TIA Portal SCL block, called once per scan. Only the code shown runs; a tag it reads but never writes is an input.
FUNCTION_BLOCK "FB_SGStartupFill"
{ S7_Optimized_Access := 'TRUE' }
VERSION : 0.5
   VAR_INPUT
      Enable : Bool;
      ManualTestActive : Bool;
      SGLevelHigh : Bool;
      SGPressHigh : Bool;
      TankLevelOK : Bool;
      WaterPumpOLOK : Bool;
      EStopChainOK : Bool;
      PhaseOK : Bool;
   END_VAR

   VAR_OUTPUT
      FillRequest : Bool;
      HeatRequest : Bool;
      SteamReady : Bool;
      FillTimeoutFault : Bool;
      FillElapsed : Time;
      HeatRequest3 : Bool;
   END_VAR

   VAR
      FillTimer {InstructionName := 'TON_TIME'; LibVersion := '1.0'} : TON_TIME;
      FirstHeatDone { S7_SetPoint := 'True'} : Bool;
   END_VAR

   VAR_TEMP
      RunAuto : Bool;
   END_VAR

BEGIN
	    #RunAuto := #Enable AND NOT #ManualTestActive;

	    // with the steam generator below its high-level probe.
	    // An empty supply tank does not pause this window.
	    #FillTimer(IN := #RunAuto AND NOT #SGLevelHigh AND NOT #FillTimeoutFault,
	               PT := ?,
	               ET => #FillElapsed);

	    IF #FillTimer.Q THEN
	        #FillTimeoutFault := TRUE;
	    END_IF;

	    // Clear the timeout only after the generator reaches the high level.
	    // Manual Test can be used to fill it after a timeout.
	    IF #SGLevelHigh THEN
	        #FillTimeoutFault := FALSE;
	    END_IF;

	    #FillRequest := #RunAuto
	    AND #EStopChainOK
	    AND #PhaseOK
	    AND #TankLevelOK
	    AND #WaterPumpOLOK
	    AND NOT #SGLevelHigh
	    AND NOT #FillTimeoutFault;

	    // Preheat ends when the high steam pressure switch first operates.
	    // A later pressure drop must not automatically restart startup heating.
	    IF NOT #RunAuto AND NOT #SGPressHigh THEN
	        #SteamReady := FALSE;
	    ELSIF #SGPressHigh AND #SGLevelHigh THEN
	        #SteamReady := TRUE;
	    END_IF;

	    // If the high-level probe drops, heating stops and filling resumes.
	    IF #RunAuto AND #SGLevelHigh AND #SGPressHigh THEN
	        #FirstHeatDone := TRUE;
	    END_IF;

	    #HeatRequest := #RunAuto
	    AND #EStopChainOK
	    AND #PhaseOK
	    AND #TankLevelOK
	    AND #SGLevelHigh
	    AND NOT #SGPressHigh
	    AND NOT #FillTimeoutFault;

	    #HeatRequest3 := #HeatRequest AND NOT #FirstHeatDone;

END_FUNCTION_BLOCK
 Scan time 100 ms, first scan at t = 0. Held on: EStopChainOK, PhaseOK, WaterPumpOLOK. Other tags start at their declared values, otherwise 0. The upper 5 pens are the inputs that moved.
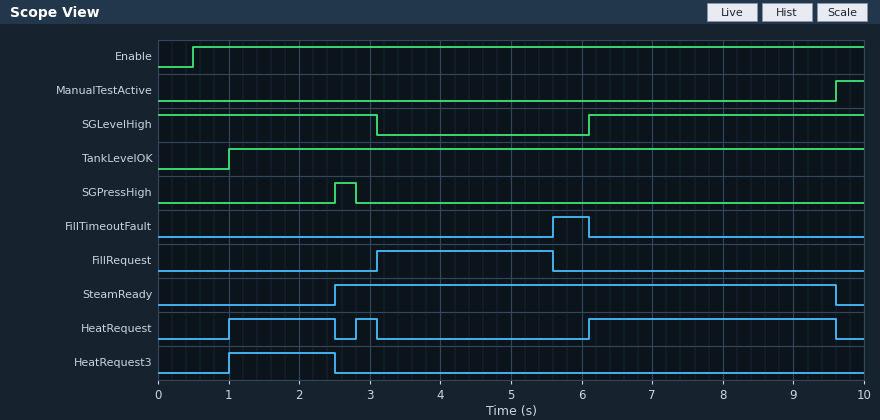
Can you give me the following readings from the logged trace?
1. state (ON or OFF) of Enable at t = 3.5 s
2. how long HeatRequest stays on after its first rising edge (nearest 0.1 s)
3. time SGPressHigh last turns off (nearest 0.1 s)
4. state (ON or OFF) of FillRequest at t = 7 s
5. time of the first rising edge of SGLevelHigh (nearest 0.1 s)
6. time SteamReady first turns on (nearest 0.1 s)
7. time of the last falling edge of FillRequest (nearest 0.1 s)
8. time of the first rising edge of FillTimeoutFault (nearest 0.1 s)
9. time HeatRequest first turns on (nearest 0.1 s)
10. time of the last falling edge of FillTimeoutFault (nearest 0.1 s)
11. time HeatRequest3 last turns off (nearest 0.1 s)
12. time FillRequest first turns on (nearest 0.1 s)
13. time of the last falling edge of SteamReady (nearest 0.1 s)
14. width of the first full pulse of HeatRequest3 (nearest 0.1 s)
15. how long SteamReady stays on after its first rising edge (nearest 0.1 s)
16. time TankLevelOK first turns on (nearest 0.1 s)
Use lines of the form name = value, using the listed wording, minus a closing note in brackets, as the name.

state (ON or OFF) of Enable at t = 3.5 s = ON
how long HeatRequest stays on after its first rising edge = 1.5 s
time SGPressHigh last turns off = 2.8 s
state (ON or OFF) of FillRequest at t = 7 s = OFF
time of the first rising edge of SGLevelHigh = 6.1 s
time SteamReady first turns on = 2.5 s
time of the last falling edge of FillRequest = 5.6 s
time of the first rising edge of FillTimeoutFault = 5.6 s
time HeatRequest first turns on = 1.0 s
time of the last falling edge of FillTimeoutFault = 6.1 s
time HeatRequest3 last turns off = 2.5 s
time FillRequest first turns on = 3.1 s
time of the last falling edge of SteamReady = 9.6 s
width of the first full pulse of HeatRequest3 = 1.5 s
how long SteamReady stays on after its first rising edge = 7.1 s
time TankLevelOK first turns on = 1.0 s
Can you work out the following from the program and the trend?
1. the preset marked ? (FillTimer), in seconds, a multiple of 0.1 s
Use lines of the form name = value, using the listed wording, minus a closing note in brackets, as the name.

the preset marked ? (FillTimer), in seconds, a multiple of 0.1 s = 2.5 s
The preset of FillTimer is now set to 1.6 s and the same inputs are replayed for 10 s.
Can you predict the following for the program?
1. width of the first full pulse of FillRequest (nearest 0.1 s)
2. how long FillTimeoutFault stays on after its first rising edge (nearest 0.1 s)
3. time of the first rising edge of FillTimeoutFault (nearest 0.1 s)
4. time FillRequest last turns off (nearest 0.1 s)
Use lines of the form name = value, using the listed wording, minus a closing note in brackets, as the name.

width of the first full pulse of FillRequest = 1.6 s
how long FillTimeoutFault stays on after its first rising edge = 1.4 s
time of the first rising edge of FillTimeoutFault = 4.7 s
time FillRequest last turns off = 4.7 s
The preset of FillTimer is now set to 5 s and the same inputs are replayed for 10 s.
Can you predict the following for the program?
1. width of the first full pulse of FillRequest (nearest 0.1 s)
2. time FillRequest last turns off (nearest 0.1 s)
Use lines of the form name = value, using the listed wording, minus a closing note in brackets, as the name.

width of the first full pulse of FillRequest = 3.0 s
time FillRequest last turns off = 6.1 s
